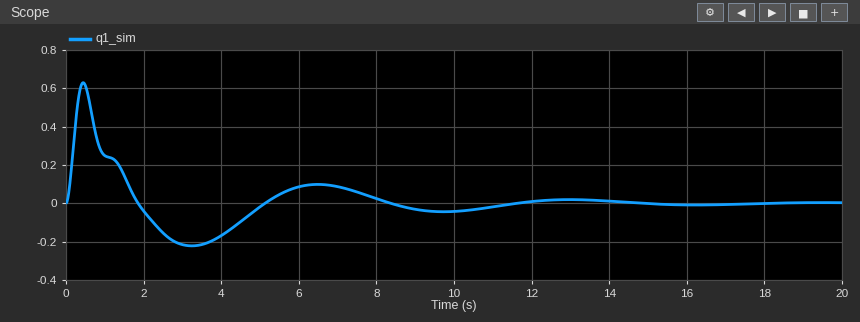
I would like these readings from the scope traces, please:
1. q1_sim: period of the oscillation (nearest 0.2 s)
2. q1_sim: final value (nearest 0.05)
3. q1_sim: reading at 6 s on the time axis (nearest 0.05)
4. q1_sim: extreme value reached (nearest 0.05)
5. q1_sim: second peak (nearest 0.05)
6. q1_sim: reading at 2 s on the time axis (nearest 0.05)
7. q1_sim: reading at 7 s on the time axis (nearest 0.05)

6.0 s
0.00
0.10
0.65
0.10
-0.05
0.10
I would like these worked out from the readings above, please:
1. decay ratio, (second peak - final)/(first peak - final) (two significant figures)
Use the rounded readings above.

0.15
